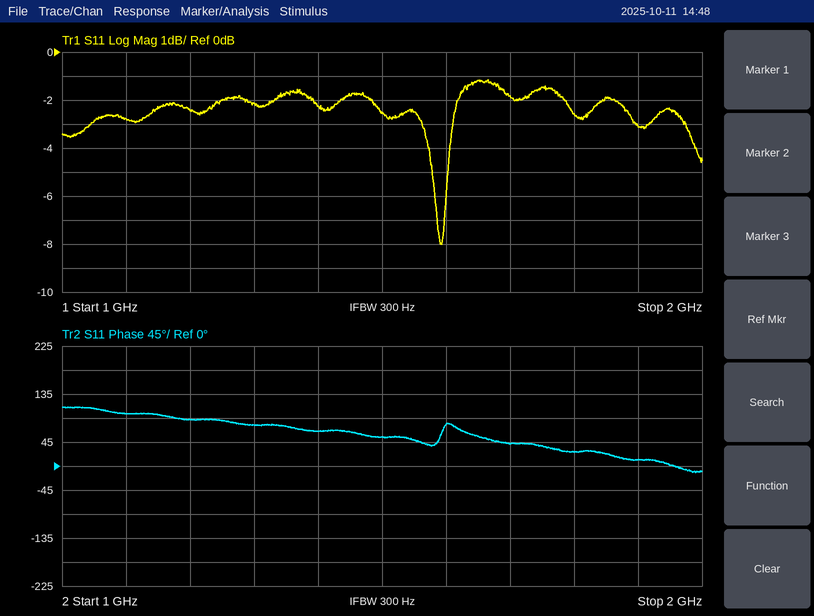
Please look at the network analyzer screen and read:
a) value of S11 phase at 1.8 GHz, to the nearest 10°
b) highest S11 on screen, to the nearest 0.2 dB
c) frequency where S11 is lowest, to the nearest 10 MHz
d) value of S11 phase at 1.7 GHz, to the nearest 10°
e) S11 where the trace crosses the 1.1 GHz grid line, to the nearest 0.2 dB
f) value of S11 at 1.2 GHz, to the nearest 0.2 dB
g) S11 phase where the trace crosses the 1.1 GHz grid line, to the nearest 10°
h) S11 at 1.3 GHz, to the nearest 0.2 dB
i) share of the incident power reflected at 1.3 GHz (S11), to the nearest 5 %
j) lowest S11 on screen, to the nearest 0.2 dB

30°
-1.2 dB
1.59 GHz
40°
-2.8 dB
-2.4 dB
100°
-2.2 dB
60 %
-8.0 dB
